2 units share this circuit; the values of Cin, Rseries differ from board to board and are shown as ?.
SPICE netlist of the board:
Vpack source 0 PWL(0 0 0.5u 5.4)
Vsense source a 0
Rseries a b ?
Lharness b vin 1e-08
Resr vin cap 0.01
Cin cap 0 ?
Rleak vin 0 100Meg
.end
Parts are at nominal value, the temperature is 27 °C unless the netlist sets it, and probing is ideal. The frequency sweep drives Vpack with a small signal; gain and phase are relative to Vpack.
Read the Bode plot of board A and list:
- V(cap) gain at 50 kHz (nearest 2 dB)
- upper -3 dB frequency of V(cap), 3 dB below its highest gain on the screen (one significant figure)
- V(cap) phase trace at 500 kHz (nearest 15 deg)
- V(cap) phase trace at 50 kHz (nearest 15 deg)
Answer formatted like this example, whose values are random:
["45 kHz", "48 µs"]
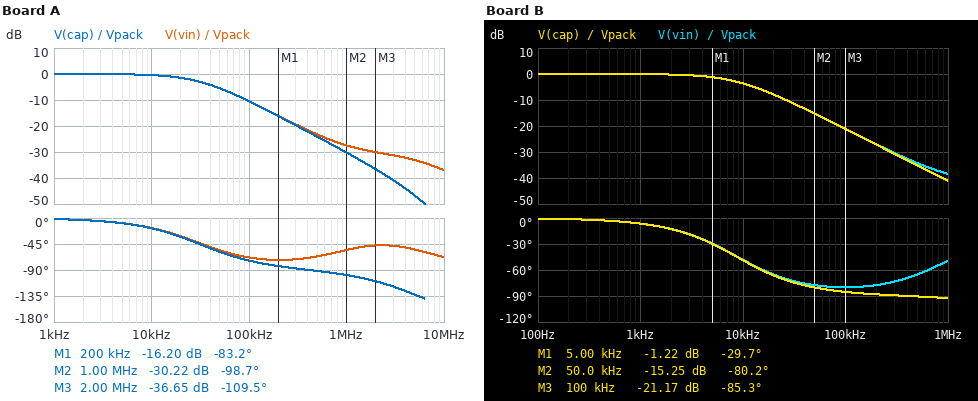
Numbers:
["-6 dB", "30 kHz", "-90 deg", "-60 deg"]
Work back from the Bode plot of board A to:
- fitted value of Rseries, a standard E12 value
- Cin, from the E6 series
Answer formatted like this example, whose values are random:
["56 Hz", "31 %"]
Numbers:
["0.33 Ω", "15 µF"]
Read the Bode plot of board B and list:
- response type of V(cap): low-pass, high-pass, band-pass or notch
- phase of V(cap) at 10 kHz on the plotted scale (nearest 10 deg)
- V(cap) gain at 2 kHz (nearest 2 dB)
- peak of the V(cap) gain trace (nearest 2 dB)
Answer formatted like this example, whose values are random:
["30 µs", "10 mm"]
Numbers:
["low-pass", "-50 deg", "0 dB", "0 dB"]
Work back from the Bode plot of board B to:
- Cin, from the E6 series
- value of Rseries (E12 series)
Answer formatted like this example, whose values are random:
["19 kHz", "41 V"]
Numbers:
["15 µF", "1.2 Ω"]
